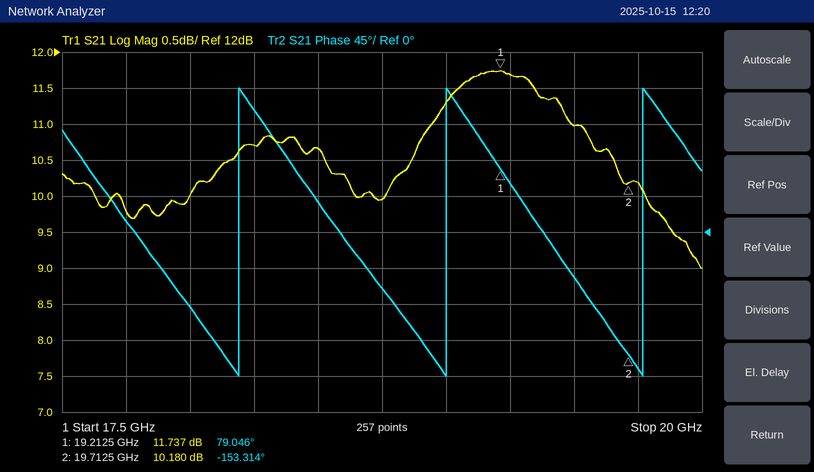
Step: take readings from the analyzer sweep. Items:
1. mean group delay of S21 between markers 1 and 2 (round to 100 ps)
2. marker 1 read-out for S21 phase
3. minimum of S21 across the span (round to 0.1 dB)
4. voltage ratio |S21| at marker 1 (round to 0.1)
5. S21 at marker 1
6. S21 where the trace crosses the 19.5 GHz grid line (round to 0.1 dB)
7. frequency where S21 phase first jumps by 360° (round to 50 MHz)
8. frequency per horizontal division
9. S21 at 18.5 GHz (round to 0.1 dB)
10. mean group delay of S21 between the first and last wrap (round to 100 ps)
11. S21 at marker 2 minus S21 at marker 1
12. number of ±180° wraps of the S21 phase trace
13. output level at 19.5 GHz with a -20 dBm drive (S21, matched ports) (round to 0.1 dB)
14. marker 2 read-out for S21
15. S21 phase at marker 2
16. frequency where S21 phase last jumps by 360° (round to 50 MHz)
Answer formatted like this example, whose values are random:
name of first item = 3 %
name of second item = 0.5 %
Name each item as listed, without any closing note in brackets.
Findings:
mean group delay of S21 between markers 1 and 2 = 1.3 ns
marker 1 read-out for S21 phase = 79.046°
minimum of S21 across the span = 9.0 dB
voltage ratio |S21| at marker 1 = 3.9
S21 at marker 1 = 11.737 dB
S21 where the trace crosses the 19.5 GHz grid line = 11.0 dB
frequency where S21 phase first jumps by 360° = 18.20 GHz
frequency per horizontal division = 250 MHz
S21 at 18.5 GHz = 10.7 dB
mean group delay of S21 between the first and last wrap = 1.3 ns
S21 at marker 2 minus S21 at marker 1 = -1.557 dB
number of ±180° wraps of the S21 phase trace = 3
output level at 19.5 GHz with a -20 dBm drive (S21, matched ports) = -9.0 dBm
marker 2 read-out for S21 = 10.180 dB
S21 phase at marker 2 = -153.314°
frequency where S21 phase last jumps by 360° = 19.75 GHz
